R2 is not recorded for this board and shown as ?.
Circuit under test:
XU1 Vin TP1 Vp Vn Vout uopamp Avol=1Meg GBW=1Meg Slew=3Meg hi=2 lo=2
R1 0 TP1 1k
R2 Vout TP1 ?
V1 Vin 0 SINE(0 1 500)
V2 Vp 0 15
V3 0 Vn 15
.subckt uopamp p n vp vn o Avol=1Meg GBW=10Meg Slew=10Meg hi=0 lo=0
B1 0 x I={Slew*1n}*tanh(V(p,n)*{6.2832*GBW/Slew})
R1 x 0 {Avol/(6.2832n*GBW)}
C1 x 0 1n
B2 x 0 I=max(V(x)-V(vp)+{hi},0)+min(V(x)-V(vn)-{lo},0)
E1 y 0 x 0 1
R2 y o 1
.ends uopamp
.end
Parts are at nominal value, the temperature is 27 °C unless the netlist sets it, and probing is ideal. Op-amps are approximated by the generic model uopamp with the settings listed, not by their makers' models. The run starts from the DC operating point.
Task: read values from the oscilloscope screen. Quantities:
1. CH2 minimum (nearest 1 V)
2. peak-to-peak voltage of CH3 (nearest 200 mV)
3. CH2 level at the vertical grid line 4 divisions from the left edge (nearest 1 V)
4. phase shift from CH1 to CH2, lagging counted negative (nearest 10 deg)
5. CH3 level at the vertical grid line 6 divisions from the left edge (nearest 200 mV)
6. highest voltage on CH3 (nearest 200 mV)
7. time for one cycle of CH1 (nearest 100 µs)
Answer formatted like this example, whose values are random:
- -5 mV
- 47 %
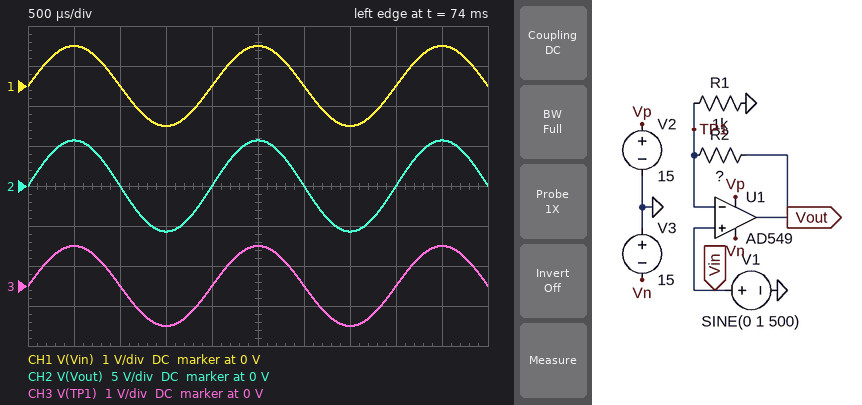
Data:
- -6 V
- 2.0 V
- 0 V
- 0 deg
- 0 V
- 1.0 V
- 2.0 ms
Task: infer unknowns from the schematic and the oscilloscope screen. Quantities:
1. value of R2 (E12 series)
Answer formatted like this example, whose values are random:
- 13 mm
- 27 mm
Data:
- 4.7 kΩ
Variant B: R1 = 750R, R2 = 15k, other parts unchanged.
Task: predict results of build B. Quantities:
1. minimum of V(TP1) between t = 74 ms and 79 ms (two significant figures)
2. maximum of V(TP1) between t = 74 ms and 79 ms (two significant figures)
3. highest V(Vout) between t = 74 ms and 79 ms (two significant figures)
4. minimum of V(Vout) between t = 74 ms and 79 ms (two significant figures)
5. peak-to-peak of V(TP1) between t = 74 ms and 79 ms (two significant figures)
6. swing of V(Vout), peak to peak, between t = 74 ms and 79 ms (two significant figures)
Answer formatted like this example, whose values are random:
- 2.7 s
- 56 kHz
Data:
- -620 mV
- 620 mV
- 13 V
- -13 V
- 1.2 V
- 26 V
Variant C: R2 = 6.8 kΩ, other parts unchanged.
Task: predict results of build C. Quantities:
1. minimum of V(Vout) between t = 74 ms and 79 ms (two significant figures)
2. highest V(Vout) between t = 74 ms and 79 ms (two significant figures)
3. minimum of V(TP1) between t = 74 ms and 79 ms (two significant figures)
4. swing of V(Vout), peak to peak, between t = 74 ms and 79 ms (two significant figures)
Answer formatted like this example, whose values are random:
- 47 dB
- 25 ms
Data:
- -7.8 V
- 7.8 V
- -1.0 V
- 16 V
